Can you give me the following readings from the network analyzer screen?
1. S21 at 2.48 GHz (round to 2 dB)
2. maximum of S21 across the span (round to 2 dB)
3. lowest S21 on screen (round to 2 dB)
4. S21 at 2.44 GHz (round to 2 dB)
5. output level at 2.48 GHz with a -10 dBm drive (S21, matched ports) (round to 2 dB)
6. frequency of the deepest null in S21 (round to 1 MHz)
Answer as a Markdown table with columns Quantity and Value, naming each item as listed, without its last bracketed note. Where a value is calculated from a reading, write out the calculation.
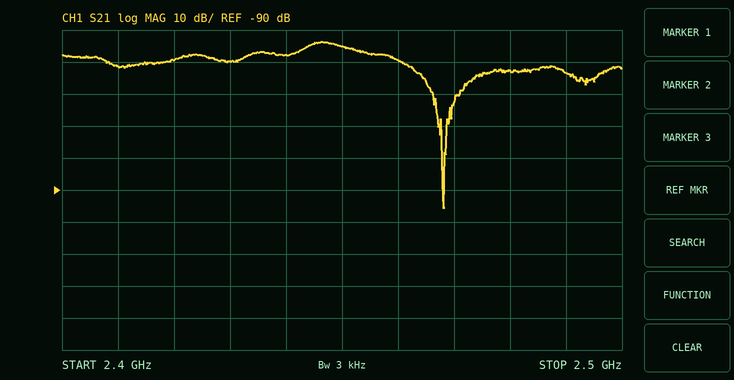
| Quantity | Value |
|---|---|
| S21 at 2.48 GHz | -52 dB |
| maximum of S21 across the span | -44 dB |
| lowest S21 on screen | -96 dB |
| S21 at 2.44 GHz | -48 dB |
| output level at 2.48 GHz with a -10 dBm drive (S21, matched ports) | -10 dBm + (-52 dB) = -62 dBm |
| frequency of the deepest null in S21 | 2.468 GHz |
